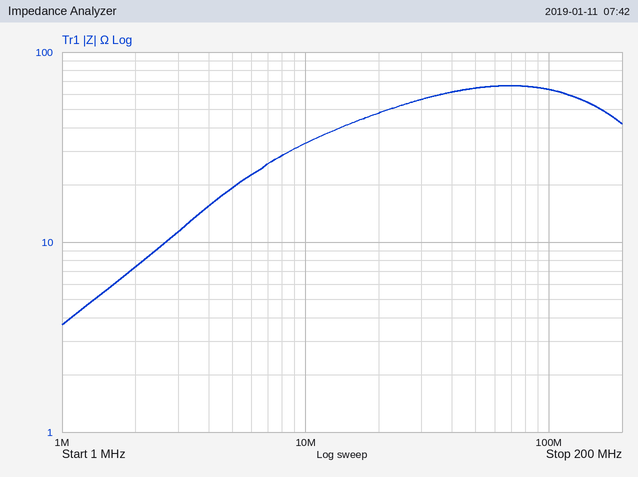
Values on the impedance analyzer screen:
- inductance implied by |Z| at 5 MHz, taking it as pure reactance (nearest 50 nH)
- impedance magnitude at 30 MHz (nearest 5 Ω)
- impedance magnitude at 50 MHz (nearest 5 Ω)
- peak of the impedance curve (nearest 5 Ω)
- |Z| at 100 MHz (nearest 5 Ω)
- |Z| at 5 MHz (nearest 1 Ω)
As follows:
600 nH
55 Ω
65 Ω
65 Ω
65 Ω
19 Ω
